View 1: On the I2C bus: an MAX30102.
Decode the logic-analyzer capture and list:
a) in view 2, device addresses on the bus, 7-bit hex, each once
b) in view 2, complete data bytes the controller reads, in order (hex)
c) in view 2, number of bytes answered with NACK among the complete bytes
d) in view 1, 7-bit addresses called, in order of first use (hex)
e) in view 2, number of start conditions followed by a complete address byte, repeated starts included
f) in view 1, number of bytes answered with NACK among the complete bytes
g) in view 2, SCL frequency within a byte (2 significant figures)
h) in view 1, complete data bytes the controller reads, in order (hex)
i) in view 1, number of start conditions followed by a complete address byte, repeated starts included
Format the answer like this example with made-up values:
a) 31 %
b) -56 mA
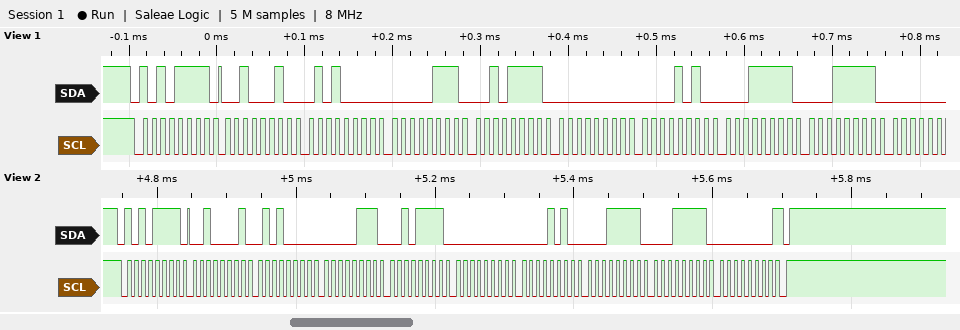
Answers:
a) 0x57
b) 21 50 07 2F 00 0A 1F 1F 00
c) 1
d) 0x57
e) 1
f) 0
g) 100 kHz
h) 22 50 07 2F 00 0A 1F 1F
i) 1
